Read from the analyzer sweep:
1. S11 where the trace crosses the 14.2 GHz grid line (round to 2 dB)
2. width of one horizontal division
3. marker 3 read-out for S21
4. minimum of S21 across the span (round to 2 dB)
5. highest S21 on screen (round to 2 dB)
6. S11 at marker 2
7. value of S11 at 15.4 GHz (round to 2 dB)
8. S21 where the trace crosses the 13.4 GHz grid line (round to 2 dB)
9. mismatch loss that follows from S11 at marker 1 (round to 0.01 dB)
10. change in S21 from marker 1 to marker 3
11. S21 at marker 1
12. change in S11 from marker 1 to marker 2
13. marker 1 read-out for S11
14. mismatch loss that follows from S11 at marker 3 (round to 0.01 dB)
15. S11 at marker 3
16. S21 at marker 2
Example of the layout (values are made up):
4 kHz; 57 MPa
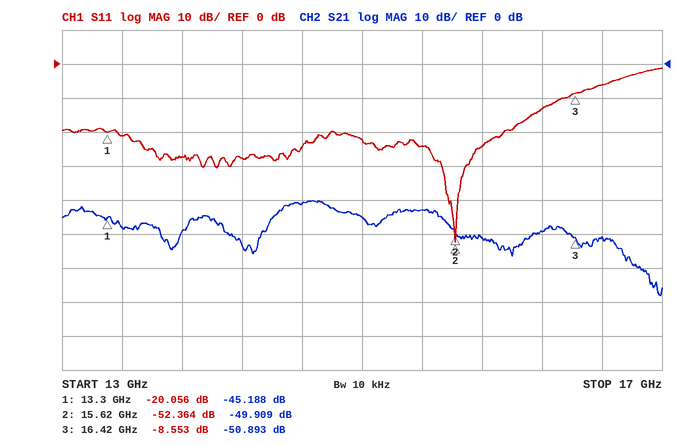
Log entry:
-28 dB; 400 MHz; -50.893 dB; -68 dB; -40 dB; -52.364 dB; -24 dB; -48 dB; 0.04 dB; -5.705 dB; -45.188 dB; -32.308 dB; -20.056 dB; 0.65 dB; -8.553 dB; -49.909 dB
